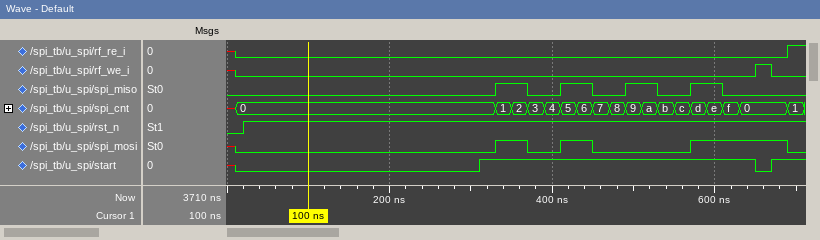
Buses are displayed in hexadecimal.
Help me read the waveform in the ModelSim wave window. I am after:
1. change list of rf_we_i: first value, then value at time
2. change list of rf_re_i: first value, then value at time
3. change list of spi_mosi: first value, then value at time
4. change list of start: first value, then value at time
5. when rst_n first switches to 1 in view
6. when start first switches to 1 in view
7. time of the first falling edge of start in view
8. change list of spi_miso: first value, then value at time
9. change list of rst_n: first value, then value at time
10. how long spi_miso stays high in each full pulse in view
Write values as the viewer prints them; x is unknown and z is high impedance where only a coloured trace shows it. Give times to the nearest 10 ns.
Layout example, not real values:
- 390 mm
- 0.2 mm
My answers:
- x, 0 at 10 ns, 1 at 650 ns, 0 at 670 ns
- x, 0 at 10 ns, 1 at 690 ns
- x, 0 at 10 ns, 1 at 330 ns, 0 at 370 ns, 1 at 410 ns, 0 at 450 ns, 1 at 570 ns, 0 at 690 ns
- x, 0 at 10 ns, 1 at 310 ns, 0 at 650 ns, 1 at 670 ns
- 20 ns
- 310 ns
- 650 ns
- 0, 1 at 330 ns, 0 at 370 ns, 1 at 410 ns, 0 at 450 ns, 1 at 490 ns, 0 at 530 ns, 1 at 570 ns, 0 at 610 ns
- 0, 1 at 20 ns
- 40 ns, 40 ns, 40 ns, 40 ns
